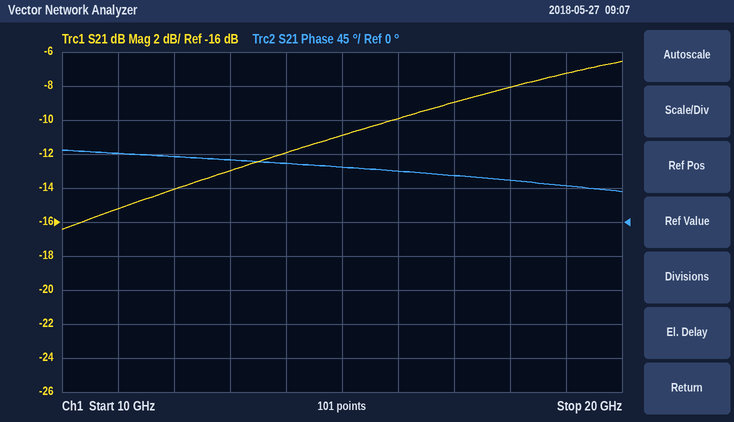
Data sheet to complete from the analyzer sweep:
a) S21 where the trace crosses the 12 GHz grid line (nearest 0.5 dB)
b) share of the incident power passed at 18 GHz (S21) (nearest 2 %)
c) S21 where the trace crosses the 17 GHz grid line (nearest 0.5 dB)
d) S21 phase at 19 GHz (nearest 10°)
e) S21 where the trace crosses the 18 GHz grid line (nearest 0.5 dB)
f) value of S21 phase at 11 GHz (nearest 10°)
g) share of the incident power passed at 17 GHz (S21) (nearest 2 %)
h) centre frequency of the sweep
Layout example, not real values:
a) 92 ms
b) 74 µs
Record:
a) -14.0 dB
b) 16 %
c) -9.0 dB
d) 50°
e) -8.0 dB
f) 90°
g) 12 %
h) 15 GHz
